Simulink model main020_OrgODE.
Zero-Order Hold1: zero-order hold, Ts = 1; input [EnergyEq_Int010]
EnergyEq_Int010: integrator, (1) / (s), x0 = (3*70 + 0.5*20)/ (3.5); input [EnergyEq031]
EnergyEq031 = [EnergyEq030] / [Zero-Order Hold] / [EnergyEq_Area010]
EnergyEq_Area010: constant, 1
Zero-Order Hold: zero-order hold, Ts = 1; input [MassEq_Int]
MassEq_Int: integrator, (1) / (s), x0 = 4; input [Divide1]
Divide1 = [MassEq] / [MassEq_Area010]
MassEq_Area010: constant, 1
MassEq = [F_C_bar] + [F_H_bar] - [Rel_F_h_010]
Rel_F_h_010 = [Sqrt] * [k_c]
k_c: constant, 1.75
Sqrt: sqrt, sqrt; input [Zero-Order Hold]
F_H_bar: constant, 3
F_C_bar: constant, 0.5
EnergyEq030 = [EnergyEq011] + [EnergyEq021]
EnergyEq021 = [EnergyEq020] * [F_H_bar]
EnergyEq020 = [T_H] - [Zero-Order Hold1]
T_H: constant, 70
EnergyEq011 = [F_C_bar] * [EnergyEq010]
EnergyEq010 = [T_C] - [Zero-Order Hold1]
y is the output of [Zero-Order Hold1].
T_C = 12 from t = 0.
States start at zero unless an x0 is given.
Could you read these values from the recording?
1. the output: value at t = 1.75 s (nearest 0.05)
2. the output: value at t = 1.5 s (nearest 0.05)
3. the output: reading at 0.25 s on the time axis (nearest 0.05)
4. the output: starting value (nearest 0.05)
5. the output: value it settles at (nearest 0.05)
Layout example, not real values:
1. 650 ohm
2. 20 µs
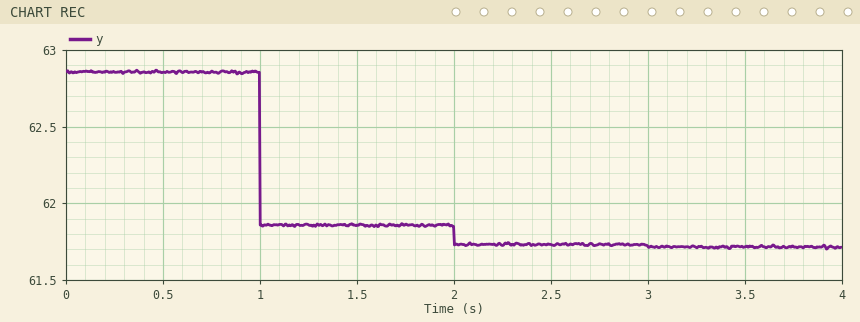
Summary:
1. 61.85
2. 61.85
3. 62.85
4. 62.85
5. 61.70
